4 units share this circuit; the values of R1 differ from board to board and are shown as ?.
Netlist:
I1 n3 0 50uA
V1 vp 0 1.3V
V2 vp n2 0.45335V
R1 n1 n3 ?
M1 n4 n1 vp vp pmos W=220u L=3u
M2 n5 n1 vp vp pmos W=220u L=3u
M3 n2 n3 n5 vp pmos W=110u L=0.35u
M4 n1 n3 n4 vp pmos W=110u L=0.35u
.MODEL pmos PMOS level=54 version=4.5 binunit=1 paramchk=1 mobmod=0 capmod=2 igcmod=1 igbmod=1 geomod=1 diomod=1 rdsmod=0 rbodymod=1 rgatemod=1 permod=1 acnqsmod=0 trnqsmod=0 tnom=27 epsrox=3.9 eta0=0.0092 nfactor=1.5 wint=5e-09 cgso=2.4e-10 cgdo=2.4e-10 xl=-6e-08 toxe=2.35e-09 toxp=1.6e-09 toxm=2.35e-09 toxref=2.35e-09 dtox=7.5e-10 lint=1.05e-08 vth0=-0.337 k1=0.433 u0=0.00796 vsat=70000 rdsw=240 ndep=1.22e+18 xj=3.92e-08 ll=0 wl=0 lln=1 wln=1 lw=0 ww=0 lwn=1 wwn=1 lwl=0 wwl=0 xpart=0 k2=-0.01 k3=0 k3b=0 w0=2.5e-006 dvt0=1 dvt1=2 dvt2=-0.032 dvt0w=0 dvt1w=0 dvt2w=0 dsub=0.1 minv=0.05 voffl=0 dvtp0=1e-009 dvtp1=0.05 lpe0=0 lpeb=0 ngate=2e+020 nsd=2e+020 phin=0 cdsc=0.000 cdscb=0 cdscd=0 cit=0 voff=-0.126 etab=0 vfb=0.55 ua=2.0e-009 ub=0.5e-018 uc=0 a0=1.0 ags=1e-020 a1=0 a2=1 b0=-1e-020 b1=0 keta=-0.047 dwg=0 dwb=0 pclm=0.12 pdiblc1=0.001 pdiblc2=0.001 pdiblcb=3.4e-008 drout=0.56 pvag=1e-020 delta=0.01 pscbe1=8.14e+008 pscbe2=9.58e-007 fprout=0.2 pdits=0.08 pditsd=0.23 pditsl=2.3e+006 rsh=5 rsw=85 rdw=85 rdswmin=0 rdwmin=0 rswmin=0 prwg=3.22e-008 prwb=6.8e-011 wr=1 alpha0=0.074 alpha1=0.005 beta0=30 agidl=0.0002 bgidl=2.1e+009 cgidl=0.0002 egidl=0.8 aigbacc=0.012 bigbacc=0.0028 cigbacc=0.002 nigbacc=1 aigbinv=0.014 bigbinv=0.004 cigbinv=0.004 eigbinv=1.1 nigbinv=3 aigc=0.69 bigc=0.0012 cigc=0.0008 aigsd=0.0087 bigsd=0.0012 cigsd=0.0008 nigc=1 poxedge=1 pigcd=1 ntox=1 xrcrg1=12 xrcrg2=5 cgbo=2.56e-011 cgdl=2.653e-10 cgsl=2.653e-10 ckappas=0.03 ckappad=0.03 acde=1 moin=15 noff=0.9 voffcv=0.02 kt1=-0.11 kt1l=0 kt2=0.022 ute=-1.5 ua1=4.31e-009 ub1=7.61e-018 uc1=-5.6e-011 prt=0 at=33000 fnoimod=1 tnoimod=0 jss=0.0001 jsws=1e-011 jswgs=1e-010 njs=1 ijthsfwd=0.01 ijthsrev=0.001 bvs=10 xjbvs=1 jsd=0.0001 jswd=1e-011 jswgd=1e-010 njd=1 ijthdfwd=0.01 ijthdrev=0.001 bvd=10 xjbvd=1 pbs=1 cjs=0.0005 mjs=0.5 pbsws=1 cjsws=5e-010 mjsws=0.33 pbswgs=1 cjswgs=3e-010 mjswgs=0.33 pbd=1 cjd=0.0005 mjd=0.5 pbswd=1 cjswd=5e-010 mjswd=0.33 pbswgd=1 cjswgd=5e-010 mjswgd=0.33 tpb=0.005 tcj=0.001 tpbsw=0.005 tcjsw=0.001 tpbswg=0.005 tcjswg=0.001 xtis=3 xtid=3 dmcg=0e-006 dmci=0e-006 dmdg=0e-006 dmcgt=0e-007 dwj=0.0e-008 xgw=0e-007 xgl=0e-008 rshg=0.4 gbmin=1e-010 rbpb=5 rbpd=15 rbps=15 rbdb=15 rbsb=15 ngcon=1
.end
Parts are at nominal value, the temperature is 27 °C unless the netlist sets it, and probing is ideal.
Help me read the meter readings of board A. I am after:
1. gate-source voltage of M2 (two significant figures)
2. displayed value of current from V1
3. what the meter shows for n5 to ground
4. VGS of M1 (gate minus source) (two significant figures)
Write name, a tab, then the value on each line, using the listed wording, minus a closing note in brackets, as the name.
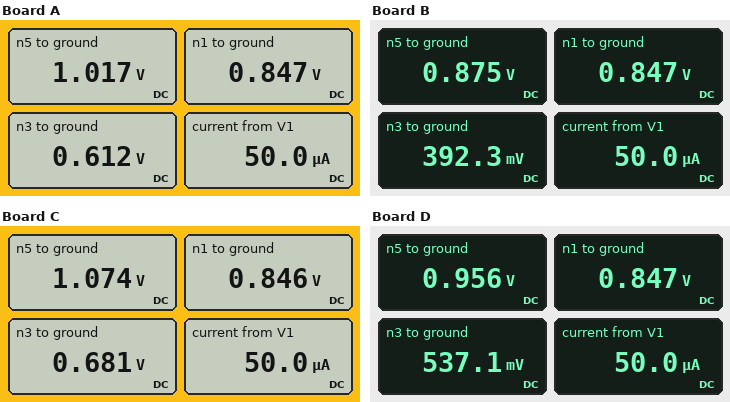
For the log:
gate-source voltage of M2	-450 mV
displayed value of current from V1	50.0 µA
what the meter shows for n5 to ground	1.017 V
VGS of M1 (gate minus source)	-450 mV
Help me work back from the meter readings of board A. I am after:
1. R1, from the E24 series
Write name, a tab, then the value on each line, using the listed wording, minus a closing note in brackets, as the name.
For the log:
R1, from the E24 series	4.7 kΩ
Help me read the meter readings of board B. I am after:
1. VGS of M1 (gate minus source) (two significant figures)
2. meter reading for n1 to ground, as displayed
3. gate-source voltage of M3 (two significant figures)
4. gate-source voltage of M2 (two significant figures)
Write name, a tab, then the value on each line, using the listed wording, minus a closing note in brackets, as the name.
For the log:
VGS of M1 (gate minus source)	-450 mV
meter reading for n1 to ground, as displayed	0.847 V
gate-source voltage of M3	-480 mV
gate-source voltage of M2	-450 mV
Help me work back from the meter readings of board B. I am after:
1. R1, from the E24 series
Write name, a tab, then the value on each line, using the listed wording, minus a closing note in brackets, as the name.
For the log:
R1, from the E24 series	9.1 kΩ
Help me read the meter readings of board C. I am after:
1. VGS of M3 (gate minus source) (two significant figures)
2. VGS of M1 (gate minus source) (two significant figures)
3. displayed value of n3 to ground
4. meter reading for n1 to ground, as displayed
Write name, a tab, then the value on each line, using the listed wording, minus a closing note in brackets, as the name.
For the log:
VGS of M3 (gate minus source)	-390 mV
VGS of M1 (gate minus source)	-450 mV
displayed value of n3 to ground	0.681 V
meter reading for n1 to ground, as displayed	0.846 V
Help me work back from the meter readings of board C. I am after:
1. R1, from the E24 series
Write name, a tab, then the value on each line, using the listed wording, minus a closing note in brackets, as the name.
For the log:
R1, from the E24 series	3.3 kΩ
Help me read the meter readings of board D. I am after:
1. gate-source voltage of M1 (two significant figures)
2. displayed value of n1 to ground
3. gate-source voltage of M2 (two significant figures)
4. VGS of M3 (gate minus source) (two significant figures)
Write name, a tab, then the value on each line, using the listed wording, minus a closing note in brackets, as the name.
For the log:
gate-source voltage of M1	-450 mV
displayed value of n1 to ground	0.847 V
gate-source voltage of M2	-450 mV
VGS of M3 (gate minus source)	-420 mV
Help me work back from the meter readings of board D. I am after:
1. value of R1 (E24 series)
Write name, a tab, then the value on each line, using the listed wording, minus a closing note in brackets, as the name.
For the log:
value of R1	6.2 kΩ
